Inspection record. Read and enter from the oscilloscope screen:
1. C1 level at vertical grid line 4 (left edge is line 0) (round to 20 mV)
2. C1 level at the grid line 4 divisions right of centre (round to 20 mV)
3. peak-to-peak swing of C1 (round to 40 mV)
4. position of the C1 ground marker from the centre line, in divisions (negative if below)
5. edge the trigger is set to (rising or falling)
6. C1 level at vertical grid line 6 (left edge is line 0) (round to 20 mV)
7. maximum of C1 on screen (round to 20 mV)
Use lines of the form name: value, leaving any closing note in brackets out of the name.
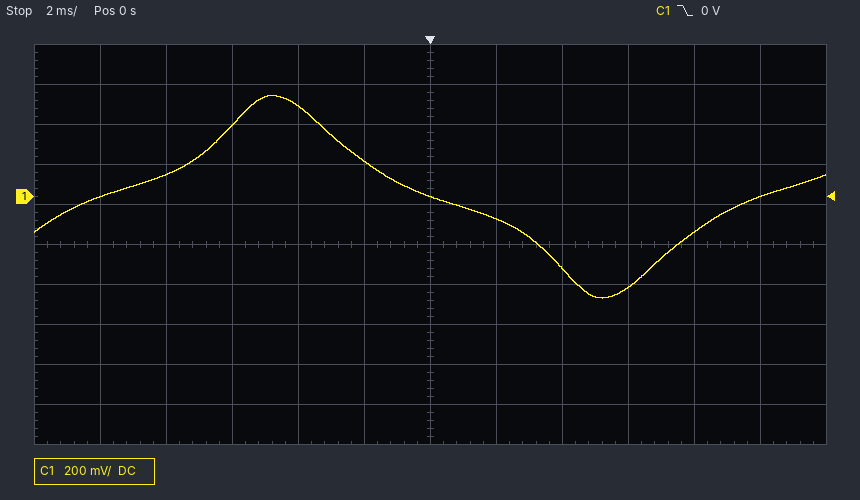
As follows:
C1 level at vertical grid line 4 (left edge is line 0): 460 mV
C1 level at the grid line 4 divisions right of centre: -180 mV
peak-to-peak swing of C1: 1.00 V
position of the C1 ground marker from the centre line, in divisions: +1.2 div
edge the trigger is set to: falling
C1 level at vertical grid line 6 (left edge is line 0): 0 mV
maximum of C1 on screen: 500 mV
